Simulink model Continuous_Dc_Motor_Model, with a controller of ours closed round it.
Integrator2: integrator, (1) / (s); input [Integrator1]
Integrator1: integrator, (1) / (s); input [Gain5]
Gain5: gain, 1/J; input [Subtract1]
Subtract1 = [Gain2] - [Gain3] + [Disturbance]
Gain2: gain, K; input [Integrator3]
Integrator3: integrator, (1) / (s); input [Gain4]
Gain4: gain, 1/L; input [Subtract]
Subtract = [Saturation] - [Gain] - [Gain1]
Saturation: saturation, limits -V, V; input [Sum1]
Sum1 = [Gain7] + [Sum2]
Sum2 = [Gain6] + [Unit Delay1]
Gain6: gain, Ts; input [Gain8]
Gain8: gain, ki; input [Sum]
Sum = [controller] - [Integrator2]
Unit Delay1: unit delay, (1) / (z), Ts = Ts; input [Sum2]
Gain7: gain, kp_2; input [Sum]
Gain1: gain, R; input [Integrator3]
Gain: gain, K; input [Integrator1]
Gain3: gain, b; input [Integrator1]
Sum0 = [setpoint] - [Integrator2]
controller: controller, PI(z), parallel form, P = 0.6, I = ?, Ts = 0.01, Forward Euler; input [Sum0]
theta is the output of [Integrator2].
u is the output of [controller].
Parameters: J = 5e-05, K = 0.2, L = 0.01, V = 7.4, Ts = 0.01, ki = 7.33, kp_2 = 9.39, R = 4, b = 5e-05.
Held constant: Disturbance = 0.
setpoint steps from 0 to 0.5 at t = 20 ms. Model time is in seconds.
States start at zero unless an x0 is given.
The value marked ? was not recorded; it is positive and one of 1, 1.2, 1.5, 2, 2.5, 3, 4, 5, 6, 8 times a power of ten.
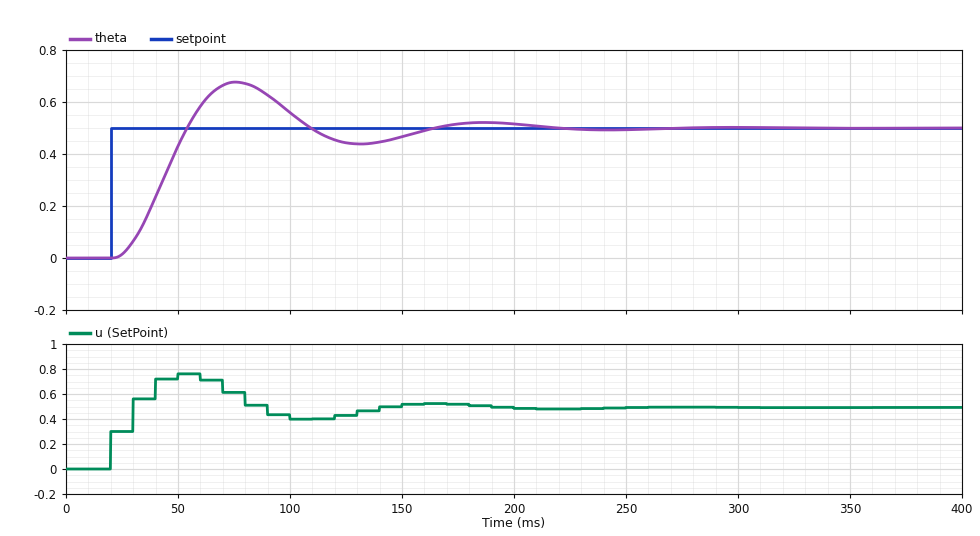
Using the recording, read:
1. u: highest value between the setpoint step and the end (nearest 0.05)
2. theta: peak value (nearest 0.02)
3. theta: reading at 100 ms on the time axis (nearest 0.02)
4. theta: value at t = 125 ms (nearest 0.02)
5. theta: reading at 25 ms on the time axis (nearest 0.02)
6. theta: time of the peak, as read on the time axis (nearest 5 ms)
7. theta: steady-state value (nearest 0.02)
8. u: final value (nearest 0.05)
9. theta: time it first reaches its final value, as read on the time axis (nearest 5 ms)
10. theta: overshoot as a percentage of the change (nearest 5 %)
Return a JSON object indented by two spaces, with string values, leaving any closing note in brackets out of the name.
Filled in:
{
  "u: highest value between the setpoint step and the end": "0.75",
  "theta: peak value": "0.68",
  "theta: reading at 100 ms on the time axis": "0.56",
  "theta: value at t = 125 ms": "0.44",
  "theta: reading at 25 ms on the time axis": "0.02",
  "theta: time of the peak, as read on the time axis": "75 ms",
  "theta: steady-state value": "0.50",
  "u: final value": "0.50",
  "theta: time it first reaches its final value, as read on the time axis": "55 ms",
  "theta: overshoot as a percentage of the change": "35 %"
}
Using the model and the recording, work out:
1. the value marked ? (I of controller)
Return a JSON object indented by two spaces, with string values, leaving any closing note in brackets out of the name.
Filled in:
{
  "the value marked ?": "60"
}
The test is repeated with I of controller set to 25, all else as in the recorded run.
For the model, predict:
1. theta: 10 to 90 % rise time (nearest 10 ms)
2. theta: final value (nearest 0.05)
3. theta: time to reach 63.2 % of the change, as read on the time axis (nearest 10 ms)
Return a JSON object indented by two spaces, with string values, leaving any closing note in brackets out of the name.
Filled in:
{
  "theta: 10 to 90 % rise time": "60 ms",
  "theta: final value": "0.50",
  "theta: time to reach 63.2 % of the change, as read on the time axis": "50 ms"
}
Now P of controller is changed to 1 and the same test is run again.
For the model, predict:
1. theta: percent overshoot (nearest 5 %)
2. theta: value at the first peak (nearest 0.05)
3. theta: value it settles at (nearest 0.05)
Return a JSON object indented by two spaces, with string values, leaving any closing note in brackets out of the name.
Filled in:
{
  "theta: percent overshoot": "20 %",
  "theta: value at the first peak": "0.60",
  "theta: value it settles at": "0.50"
}
